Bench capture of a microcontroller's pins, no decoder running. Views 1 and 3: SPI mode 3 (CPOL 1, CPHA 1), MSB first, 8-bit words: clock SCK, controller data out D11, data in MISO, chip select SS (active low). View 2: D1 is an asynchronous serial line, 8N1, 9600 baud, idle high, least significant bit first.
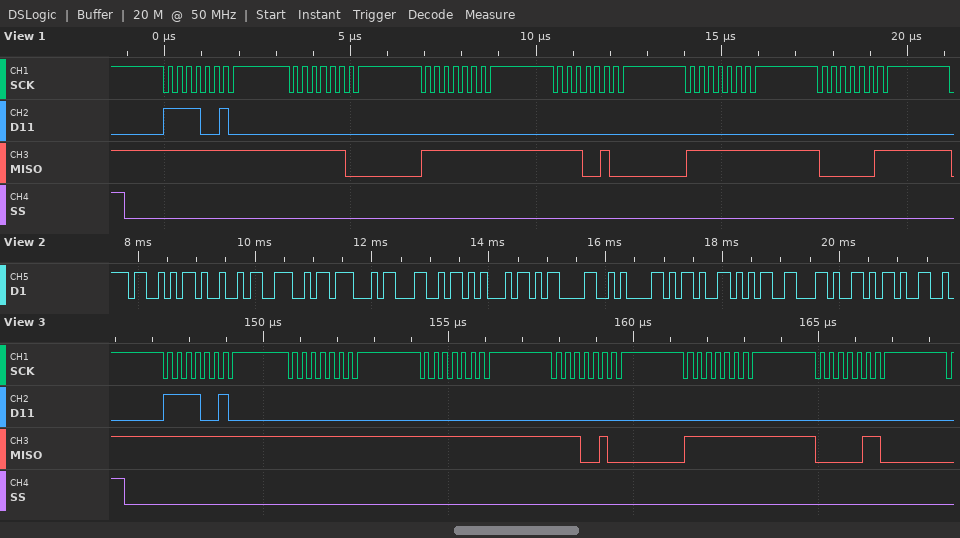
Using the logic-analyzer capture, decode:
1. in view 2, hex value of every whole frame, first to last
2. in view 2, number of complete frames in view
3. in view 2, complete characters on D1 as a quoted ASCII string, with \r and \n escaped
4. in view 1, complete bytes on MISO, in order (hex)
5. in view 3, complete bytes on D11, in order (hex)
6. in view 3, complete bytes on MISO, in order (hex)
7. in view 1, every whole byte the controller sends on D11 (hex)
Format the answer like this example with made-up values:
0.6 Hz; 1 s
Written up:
53 49 4E 47 4C 45 0D 0A 2D 35 2C 2D; 12; "SINGLE\r\n-5,-"; FF FC FF E4 FF 03; 0xF2 0x00 0x00 0x00 0x00 0x00; 0xFF 0xFF 0xFF 0xE4 0xFF 0x06; F2 00 00 00 00 00
